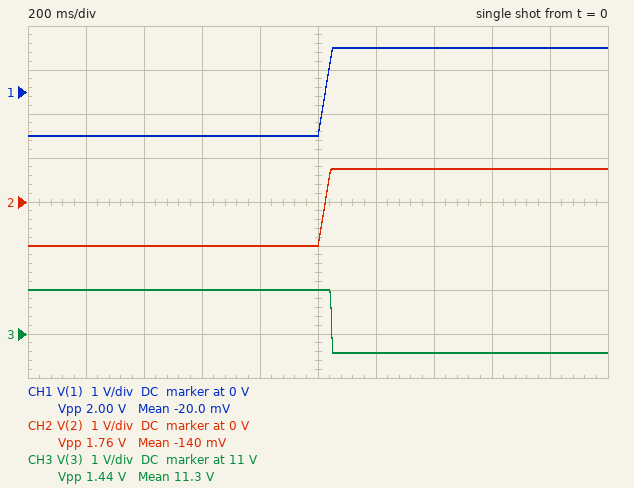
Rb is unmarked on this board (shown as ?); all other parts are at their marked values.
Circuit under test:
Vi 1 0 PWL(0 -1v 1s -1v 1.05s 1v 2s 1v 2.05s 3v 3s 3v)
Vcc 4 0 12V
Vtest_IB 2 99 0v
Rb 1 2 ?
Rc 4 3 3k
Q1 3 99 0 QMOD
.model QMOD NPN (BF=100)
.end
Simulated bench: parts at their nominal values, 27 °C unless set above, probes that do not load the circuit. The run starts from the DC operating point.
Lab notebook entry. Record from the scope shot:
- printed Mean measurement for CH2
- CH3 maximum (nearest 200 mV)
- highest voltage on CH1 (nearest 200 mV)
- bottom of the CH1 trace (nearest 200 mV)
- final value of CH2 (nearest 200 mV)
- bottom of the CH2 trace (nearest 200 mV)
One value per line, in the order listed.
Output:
-140 mV
12.0 V
1.0 V
-1.0 V
800 mV
-1.0 V
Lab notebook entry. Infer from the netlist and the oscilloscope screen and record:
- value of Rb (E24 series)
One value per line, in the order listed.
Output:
51 kΩ
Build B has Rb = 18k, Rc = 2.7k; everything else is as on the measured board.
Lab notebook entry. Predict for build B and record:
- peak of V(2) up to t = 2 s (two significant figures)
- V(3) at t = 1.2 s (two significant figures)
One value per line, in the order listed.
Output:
780 mV
8.7 V
